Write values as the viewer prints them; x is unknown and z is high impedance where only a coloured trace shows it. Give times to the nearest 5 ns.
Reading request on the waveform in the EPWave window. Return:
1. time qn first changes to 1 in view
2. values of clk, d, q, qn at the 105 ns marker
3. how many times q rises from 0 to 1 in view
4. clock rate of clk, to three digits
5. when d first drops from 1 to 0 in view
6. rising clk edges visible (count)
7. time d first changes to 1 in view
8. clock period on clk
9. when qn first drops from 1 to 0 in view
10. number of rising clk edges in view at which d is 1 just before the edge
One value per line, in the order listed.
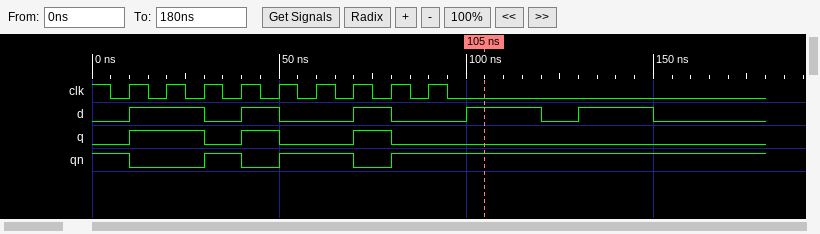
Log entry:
30 ns
clk=0, d=1, q=0, qn=1
3
100 MHz
30 ns
9
10 ns
10 ns
10 ns
4
